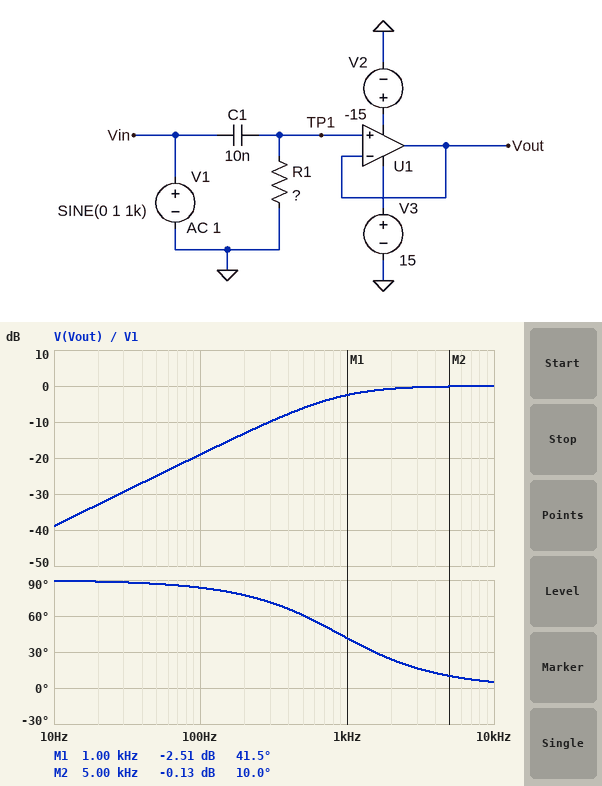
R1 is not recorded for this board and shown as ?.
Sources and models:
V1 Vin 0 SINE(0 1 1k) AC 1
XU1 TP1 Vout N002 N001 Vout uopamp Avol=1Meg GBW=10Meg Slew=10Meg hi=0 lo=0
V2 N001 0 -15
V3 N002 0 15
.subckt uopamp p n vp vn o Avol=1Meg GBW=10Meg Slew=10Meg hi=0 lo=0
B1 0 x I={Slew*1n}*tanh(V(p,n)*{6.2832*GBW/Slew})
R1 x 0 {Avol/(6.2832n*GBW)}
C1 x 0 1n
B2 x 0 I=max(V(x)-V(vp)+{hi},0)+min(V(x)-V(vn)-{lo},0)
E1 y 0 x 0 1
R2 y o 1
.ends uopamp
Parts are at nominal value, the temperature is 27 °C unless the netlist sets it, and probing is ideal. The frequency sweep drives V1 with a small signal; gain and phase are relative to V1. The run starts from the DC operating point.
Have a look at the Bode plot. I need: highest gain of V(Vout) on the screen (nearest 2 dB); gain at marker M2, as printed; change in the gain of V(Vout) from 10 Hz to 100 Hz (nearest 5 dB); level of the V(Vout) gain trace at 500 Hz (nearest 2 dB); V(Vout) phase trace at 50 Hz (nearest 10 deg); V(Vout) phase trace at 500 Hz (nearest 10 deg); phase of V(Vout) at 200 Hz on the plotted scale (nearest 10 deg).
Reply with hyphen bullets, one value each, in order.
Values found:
- 0 dB
- -0.13 dB
- 20 dB
- -6 dB
- 90 deg
- 60 deg
- 80 deg
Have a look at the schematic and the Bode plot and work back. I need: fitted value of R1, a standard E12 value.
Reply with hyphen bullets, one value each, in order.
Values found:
- 18 kΩ
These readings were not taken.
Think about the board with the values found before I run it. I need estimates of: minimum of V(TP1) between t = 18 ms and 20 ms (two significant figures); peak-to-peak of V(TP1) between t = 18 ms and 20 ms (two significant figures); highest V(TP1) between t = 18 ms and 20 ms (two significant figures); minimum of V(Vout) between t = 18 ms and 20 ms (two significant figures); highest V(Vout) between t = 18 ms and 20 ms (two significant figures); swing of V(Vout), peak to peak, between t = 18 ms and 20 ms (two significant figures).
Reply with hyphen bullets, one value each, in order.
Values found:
- -750 mV
- 1.5 V
- 750 mV
- -750 mV
- 750 mV
- 1.5 V
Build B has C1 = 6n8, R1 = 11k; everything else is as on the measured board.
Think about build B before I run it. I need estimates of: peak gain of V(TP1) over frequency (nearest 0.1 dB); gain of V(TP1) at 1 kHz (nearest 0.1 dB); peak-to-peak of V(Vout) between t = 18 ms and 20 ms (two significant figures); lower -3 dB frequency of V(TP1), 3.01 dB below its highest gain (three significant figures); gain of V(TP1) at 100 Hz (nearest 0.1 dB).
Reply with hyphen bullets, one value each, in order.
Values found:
- 0 dB
- -7.4 dB
- 850 mV
- 2.13 kHz
- -26.6 dB
